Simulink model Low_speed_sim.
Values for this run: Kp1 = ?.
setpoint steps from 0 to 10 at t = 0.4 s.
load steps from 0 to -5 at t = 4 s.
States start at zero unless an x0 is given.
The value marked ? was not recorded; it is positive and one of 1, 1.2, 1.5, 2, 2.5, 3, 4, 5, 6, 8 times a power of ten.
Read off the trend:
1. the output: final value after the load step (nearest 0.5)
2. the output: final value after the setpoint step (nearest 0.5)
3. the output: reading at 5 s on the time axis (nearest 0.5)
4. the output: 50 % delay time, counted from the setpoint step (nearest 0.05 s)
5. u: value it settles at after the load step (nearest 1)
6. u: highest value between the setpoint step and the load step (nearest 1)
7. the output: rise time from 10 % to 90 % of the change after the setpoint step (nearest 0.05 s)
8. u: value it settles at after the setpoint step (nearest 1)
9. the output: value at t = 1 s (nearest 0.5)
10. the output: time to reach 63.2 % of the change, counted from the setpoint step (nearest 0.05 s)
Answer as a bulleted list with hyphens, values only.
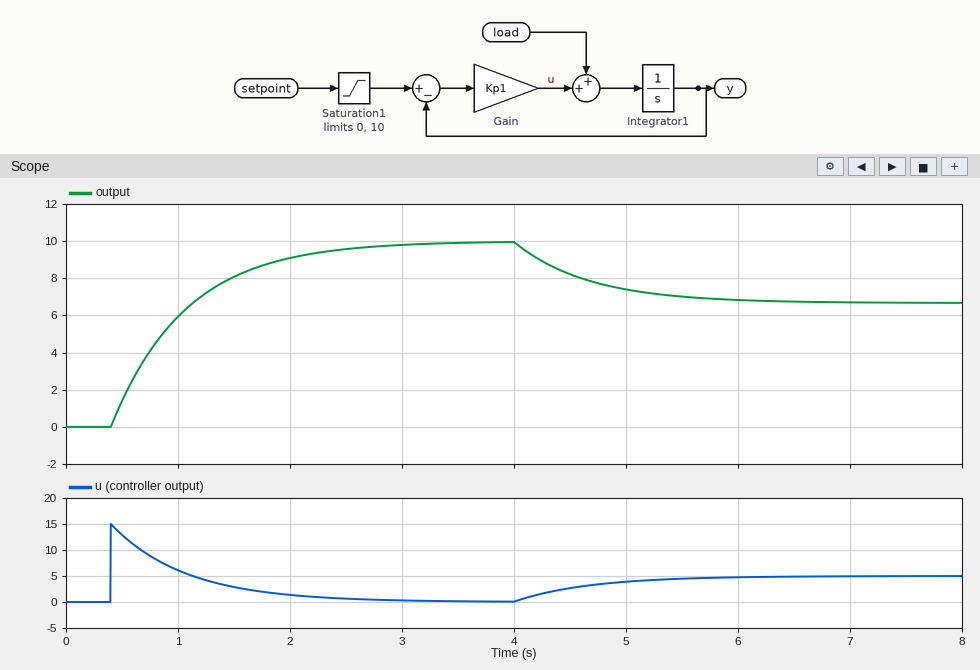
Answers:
- 6.5
- 10.0
- 7.5
- 0.45 s
- 5
- 15
- 1.45 s
- 0
- 6.0
- 0.65 s
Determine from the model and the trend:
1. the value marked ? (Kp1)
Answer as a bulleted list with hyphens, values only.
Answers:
- 1.5
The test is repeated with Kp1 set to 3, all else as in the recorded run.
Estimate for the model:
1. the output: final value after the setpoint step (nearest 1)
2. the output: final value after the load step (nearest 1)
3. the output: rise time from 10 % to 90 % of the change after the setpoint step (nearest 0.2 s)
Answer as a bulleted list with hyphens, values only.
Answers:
- 10
- 8
- 0.8 s
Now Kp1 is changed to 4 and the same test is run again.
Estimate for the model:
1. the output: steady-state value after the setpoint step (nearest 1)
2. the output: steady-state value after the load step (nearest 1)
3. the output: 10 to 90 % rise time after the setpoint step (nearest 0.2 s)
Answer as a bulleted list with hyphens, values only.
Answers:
- 10
- 9
- 0.6 s
